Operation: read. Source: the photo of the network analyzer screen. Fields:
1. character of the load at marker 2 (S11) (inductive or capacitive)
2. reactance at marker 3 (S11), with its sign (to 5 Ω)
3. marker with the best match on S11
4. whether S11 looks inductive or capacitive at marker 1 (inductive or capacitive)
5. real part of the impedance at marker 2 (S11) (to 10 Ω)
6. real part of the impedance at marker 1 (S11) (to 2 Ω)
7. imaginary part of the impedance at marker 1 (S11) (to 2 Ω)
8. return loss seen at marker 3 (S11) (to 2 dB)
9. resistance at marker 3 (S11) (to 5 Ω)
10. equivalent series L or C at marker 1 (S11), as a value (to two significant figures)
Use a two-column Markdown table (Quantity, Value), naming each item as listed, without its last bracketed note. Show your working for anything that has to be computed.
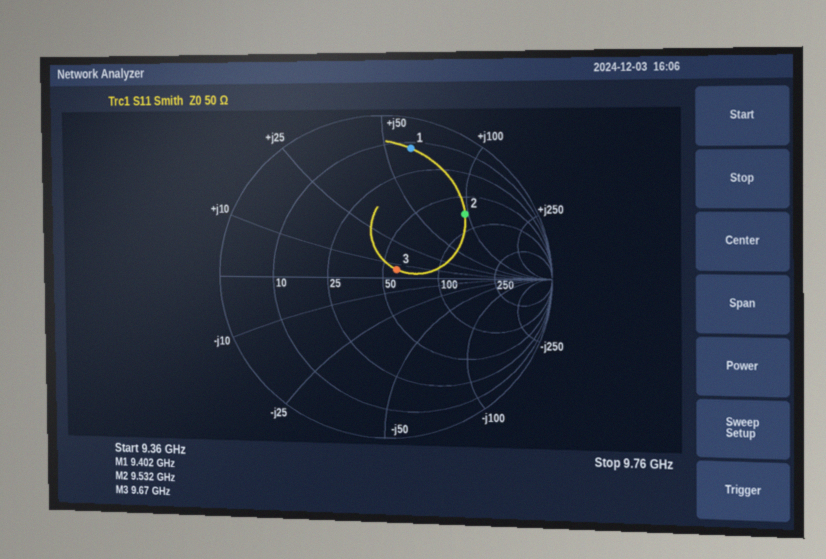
| Quantity | Value |
|---|---|
| character of the load at marker 2 (S11) | inductive |
| reactance at marker 3 (S11), with its sign | +5 Ω |
| marker with the best match on S11 | marker 3 |
| whether S11 looks inductive or capacitive at marker 1 | inductive |
| real part of the impedance at marker 2 (S11) | 70 Ω |
| real part of the impedance at marker 1 (S11) | 12 Ω |
| imaginary part of the impedance at marker 1 (S11) | +60 Ω |
| return loss seen at marker 3 (S11) | 20 dB |
| resistance at marker 3 (S11) | 60 Ω |
| equivalent series L or C at marker 1 (S11), as a value | L = 60 Ω/(2π × 9.402 GHz) ≈ 1.0 nH |
